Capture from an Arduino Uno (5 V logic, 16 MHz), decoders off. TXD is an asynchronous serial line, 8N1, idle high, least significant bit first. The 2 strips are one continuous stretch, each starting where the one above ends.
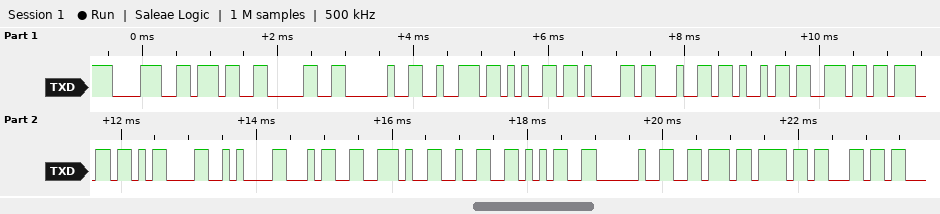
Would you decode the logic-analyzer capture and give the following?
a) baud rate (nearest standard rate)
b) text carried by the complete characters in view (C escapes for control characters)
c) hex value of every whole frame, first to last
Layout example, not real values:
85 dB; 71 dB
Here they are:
9600 baud; "870 reading\r\n4.25 vol"; 0x38 0x37 0x30 0x20 0x72 0x65 0x61 0x64 0x69 0x6E 0x67 0x0D 0x0A 0x34 0x2E 0x32 0x35 0x20 0x76 0x6F 0x6C
